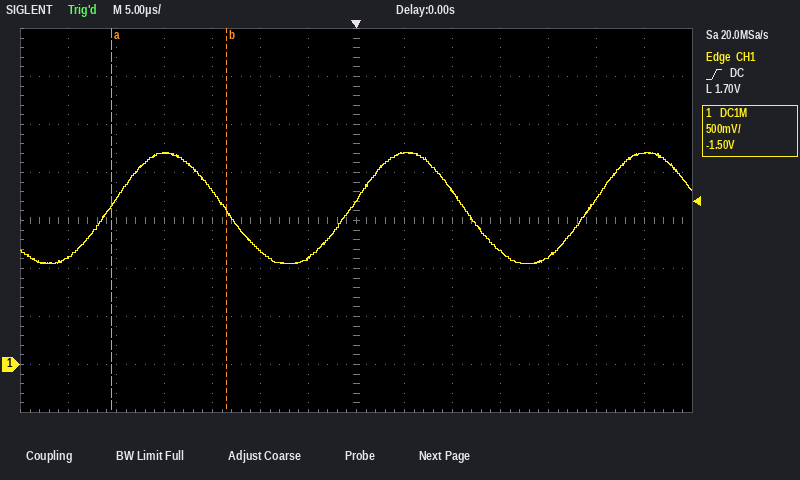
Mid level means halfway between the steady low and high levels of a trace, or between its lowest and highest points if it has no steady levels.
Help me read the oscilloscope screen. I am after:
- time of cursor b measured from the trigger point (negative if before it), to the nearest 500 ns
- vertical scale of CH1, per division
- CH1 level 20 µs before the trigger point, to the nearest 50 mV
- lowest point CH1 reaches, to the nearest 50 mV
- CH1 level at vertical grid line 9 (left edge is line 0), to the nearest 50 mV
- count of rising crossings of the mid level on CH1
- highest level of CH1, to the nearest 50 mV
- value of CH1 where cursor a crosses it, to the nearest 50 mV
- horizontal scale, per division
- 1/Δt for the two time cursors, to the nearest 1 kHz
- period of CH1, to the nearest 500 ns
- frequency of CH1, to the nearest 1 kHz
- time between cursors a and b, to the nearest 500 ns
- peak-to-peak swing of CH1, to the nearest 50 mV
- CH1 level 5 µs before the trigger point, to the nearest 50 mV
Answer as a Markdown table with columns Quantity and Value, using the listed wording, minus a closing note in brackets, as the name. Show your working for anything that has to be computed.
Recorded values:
| Quantity | Value |
|---|---|
| time of cursor b measured from the trigger point (negative if before it), to the nearest 500 ns | -13.5 µs |
| vertical scale of CH1, per division | 500 mV |
| CH1 level 20 µs before the trigger point, to the nearest 50 mV | 2.20 V |
| lowest point CH1 reaches, to the nearest 50 mV | 1.05 V |
| CH1 level at vertical grid line 9 (left edge is line 0), to the nearest 50 mV | 1.80 V |
| count of rising crossings of the mid level on CH1 | 3 |
| highest level of CH1, to the nearest 50 mV | 2.20 V |
| value of CH1 where cursor a crosses it, to the nearest 50 mV | 1.65 V |
| horizontal scale, per division | 5 µs |
| 1/Δt for the two time cursors, to the nearest 1 kHz | 1 / 12.0 µs ≈ 83 kHz |
| period of CH1, to the nearest 500 ns | 25.0 µs |
| frequency of CH1, to the nearest 1 kHz | 1 / 25.0 µs ≈ 40 kHz |
| time between cursors a and b, to the nearest 500 ns | 12.0 µs |
| peak-to-peak swing of CH1, to the nearest 50 mV | 2.20 V − (1.05 V) = 1.15 V |
| CH1 level 5 µs before the trigger point, to the nearest 50 mV | 1.10 V |
